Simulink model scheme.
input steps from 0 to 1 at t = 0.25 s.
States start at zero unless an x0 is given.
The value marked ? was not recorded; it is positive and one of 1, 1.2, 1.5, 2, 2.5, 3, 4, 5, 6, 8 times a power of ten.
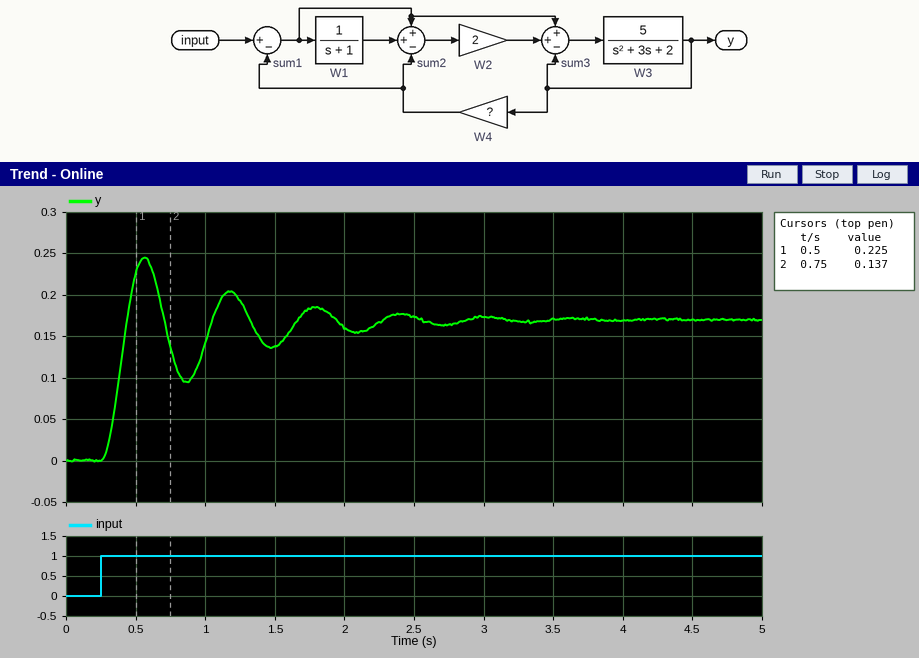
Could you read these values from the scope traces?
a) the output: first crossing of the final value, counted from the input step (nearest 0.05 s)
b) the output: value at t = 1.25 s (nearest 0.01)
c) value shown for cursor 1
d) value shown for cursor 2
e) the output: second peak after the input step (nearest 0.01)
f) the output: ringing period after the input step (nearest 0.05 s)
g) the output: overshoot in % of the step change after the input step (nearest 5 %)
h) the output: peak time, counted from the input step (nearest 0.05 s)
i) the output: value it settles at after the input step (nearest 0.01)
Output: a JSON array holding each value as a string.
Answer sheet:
["0.20 s", "0.19", "0.225", "0.137", "0.20", "0.60 s", "45 %", "0.30 s", "0.17"]
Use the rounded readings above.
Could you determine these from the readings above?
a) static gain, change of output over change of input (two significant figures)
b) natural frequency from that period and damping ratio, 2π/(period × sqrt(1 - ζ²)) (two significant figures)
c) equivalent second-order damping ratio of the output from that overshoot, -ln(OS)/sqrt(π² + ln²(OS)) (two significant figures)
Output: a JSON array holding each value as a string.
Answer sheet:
["0.17", "11 rad/s", "0.25"]
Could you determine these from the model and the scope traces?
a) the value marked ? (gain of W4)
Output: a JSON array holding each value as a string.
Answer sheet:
["4"]
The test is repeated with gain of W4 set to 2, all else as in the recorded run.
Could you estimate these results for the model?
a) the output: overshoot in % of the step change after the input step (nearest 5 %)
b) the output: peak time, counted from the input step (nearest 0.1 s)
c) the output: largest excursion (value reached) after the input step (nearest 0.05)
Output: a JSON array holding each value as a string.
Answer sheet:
["35 %", "0.4 s", "0.45"]
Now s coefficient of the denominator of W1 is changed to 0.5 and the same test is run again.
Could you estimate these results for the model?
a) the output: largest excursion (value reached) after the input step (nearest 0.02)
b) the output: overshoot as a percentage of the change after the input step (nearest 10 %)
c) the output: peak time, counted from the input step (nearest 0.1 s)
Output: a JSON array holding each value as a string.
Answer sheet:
["0.26", "50 %", "0.3 s"]
